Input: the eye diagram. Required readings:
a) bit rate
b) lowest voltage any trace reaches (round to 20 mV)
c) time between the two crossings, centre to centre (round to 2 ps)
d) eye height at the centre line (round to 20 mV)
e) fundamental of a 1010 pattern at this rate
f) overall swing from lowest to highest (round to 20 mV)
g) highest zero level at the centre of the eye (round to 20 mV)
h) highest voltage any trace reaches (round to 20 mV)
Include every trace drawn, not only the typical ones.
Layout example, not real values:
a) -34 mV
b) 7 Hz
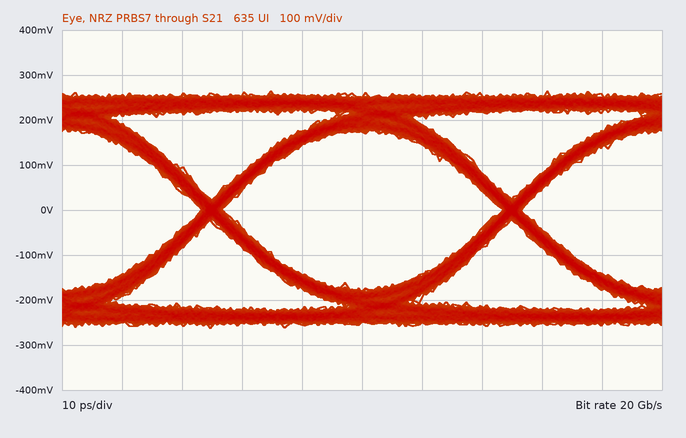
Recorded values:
a) 20 Gb/s
b) -260 mV
c) 50 ps
d) 360 mV
e) 10 GHz
f) 520 mV
g) -180 mV
h) 260 mV
